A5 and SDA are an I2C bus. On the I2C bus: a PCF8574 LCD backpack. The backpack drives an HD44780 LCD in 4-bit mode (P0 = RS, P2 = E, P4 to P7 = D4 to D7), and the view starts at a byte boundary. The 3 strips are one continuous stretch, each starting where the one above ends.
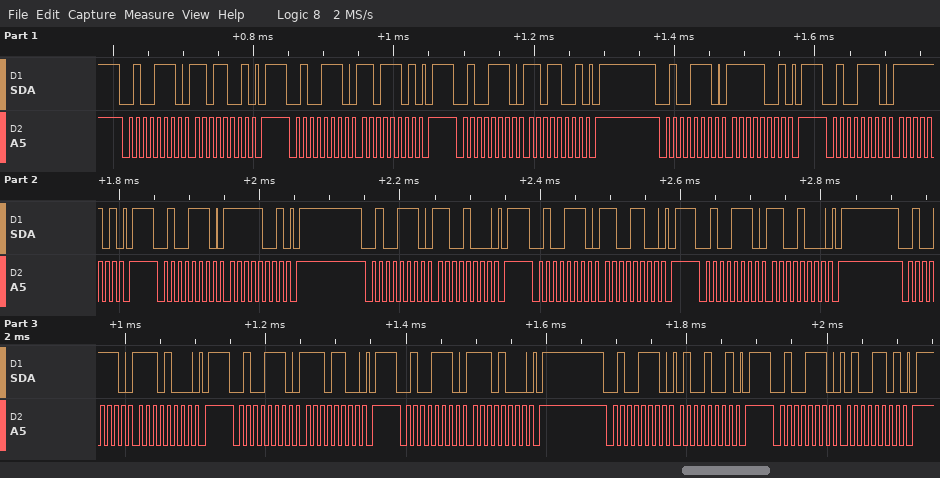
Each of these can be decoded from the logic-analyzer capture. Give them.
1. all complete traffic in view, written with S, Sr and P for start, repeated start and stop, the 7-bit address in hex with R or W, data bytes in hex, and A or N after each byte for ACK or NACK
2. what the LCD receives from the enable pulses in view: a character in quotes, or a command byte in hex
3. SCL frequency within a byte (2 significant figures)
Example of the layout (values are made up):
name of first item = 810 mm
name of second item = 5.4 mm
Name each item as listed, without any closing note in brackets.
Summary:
all complete traffic in view, written with S, Sr and P for start, repeated start and stop, the 7-bit address in hex with R or W, data bytes in hex, and A or N after each byte for ACK or NACK = S 27W A D9 A P S 27W A DD A P S 27W A D9 A P S 27W A F9 A P S 27W A FD A P S 27W A F9 A P S 27W A C8 A P S 27W A CC A P S 27W A C8 A P S 27W A E8 A P S 27W A EC A P S 27W A E8 A P S 27W A 49 A P S 27W A 4D A P
what the LCD receives from the enable pulses in view: a character in quotes, or a command byte in hex = data 0xDF 0xCE
SCL frequency within a byte = 100 kHz
